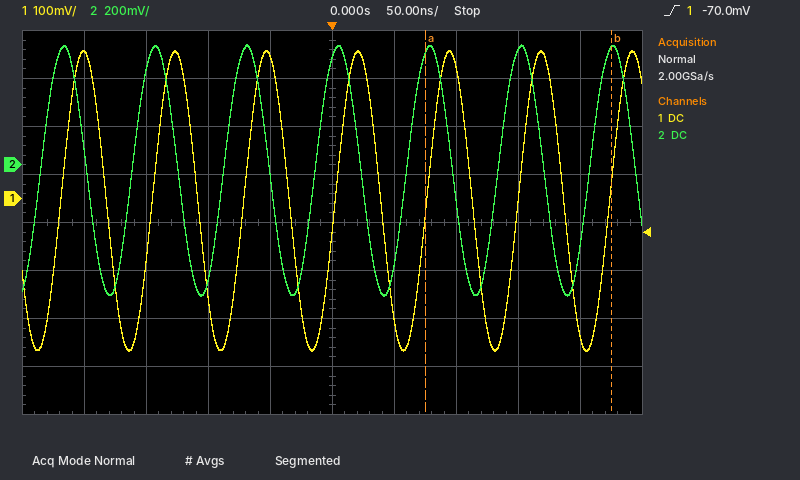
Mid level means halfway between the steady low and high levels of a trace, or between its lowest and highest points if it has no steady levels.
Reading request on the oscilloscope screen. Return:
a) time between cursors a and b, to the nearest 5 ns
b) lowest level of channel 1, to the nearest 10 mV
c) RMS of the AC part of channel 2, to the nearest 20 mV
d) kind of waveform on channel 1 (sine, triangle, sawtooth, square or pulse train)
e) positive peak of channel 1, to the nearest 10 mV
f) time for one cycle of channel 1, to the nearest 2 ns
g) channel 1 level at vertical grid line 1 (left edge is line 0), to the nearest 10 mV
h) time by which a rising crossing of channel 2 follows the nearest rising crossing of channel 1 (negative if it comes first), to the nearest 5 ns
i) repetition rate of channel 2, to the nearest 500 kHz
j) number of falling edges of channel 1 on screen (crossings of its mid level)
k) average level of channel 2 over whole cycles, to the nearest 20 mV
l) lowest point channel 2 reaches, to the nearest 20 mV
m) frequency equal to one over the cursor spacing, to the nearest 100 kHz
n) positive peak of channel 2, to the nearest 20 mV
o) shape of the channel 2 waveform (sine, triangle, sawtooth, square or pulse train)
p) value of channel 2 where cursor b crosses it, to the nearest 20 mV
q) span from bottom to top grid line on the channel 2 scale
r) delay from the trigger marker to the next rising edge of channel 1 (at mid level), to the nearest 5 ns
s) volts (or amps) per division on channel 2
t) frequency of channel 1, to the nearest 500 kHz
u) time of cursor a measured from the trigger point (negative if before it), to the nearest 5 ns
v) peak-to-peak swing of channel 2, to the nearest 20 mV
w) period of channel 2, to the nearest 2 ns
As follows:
150 ns
-320 mV
360 mV
sine
310 mV
74 ns
300 mV
-15 ns
13.5 MHz
6
-20 mV
-540 mV
6.7 MHz
500 mV
sine
480 mV
1.6 V
75 ns
200 mV
13.5 MHz
+75 ns
1.04 V
74 ns
